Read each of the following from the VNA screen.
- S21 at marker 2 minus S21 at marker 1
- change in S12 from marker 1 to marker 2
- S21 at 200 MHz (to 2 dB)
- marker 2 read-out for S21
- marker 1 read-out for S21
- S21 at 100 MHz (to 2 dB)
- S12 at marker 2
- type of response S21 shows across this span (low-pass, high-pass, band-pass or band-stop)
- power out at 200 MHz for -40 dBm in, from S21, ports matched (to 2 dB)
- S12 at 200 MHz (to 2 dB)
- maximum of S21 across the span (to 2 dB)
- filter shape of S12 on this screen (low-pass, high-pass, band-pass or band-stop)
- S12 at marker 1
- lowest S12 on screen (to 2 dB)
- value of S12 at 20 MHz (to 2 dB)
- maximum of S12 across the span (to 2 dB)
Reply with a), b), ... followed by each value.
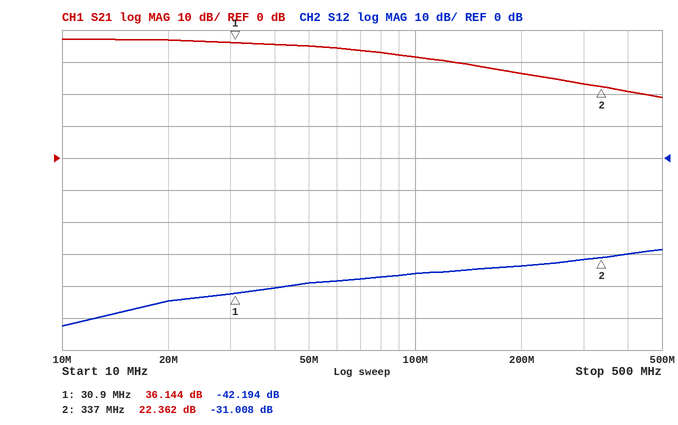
a) -13.782 dB
b) 11.186 dB
c) 26 dB
d) 22.362 dB
e) 36.144 dB
f) 32 dB
g) -31.008 dB
h) low-pass
i) -14 dBm
j) -34 dB
k) 38 dB
l) high-pass
m) -42.194 dB
n) -52 dB
o) -44 dB
p) -28 dB
